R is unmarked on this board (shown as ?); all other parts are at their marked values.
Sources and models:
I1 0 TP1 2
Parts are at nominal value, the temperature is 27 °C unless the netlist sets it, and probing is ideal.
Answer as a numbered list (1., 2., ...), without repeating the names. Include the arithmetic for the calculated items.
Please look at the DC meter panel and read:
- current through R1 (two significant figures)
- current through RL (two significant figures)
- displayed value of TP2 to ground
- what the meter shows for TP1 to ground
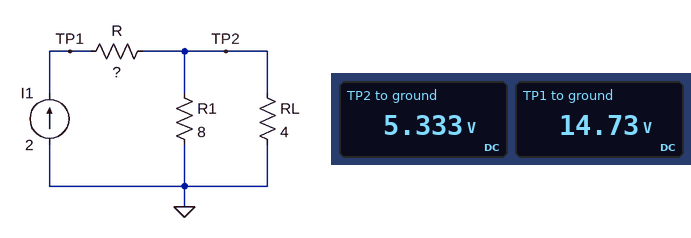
1. (5.333 V) / 8 Ω = 670 mA
2. (5.333 V) / 4 Ω = 1.3 A
3. 5.333 V
4. 14.73 V
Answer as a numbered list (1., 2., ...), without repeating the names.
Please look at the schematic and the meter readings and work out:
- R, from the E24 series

1. 4.7 Ω
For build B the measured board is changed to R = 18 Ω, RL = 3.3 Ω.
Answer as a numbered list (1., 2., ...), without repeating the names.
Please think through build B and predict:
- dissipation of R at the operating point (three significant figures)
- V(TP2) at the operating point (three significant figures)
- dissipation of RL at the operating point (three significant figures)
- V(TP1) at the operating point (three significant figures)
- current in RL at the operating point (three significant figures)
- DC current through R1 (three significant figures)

1. 72.0 W
2. 4.67 V
3. 6.62 W
4. 40.7 V
5. 1.42 A
6. 584 mA
